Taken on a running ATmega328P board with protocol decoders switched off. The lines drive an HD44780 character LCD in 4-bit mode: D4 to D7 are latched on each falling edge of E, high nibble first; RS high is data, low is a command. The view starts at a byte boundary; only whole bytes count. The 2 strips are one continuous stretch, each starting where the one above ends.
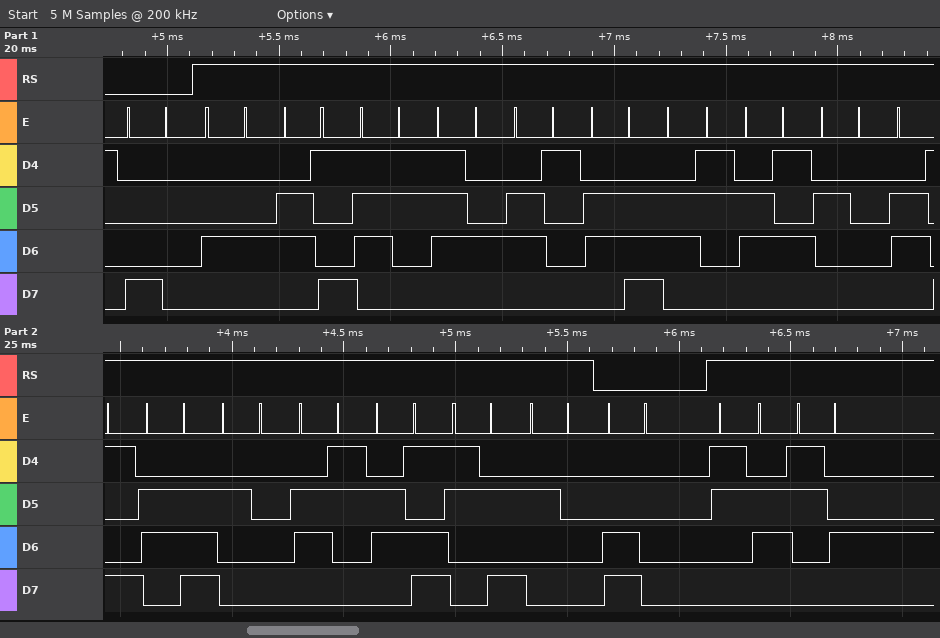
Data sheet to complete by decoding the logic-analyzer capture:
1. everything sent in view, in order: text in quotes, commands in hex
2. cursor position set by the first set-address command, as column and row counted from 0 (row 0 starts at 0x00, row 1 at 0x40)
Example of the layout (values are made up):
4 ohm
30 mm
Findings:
0x80 "Distance in cm: " 0xC0 "64"
column 0, row 0
